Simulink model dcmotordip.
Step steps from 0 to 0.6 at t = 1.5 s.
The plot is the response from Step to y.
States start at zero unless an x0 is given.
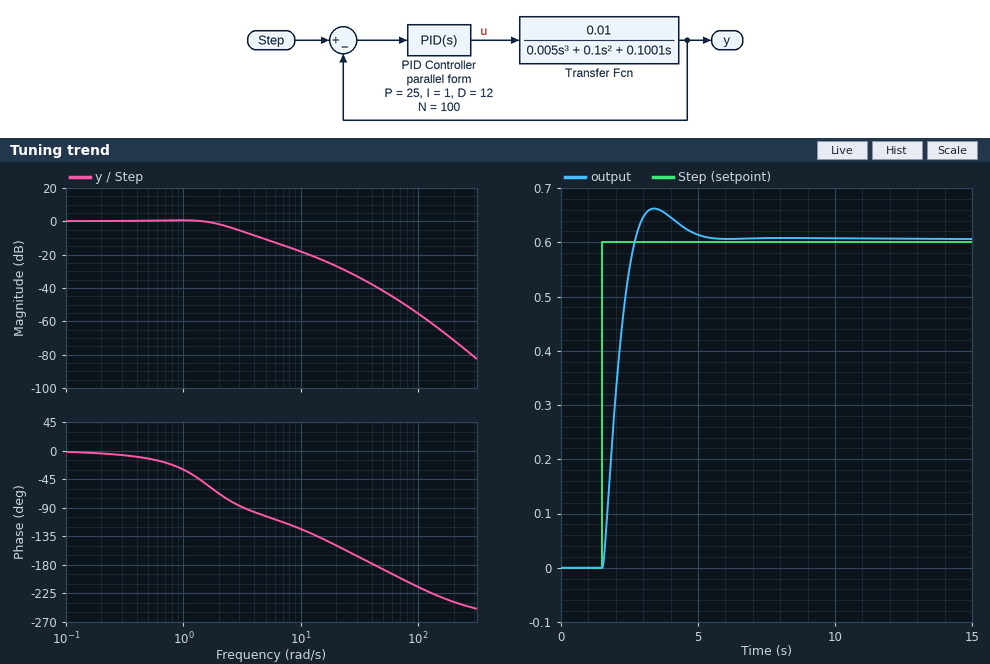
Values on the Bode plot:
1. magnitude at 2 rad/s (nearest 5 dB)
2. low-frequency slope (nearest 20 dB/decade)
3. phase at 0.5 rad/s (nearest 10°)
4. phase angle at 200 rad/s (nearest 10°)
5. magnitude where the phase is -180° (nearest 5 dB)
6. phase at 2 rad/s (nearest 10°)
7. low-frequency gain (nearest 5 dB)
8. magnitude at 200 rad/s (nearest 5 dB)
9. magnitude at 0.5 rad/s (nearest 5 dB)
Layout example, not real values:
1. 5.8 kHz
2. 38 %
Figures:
1. 0 dB
2. 0 dB/decade
3. -10°
4. -240°
5. -40 dB
6. -70°
7. 0 dB
8. -70 dB
9. 0 dB
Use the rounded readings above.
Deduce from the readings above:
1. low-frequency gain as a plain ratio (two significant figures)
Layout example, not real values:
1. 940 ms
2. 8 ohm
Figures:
1. 1.0
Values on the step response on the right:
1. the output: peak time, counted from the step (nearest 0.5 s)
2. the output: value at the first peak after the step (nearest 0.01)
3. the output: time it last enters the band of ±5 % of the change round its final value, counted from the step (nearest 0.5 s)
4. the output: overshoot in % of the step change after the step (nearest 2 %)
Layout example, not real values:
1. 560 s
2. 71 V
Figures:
1. 2.0 s
2. 0.66
3. 3.0 s
4. 10 %
